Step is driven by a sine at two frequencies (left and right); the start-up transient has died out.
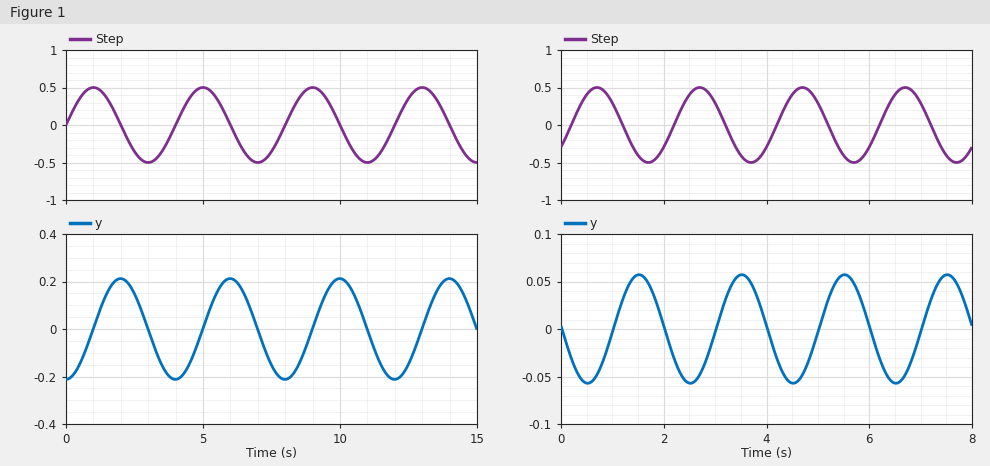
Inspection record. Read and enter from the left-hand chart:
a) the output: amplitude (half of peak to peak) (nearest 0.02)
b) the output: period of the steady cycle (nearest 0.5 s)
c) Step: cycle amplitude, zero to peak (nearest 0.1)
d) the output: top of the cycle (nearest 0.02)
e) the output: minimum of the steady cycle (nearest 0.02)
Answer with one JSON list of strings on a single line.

["0.22", "4.0 s", "0.5", "0.22", "-0.22"]
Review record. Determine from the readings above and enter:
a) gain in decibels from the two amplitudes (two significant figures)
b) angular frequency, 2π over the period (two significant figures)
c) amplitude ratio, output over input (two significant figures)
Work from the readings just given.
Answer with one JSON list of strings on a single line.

["-7.1 dB", "1.6 rad/s", "0.44"]
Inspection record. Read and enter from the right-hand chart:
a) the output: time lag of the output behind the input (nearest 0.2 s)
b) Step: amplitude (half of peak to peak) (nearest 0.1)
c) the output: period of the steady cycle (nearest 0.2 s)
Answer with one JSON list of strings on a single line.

["0.8 s", "0.5", "2.0 s"]
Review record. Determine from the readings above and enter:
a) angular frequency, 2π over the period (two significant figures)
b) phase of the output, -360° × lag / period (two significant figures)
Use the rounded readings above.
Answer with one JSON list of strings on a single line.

["3.1 rad/s", "-140°"]
